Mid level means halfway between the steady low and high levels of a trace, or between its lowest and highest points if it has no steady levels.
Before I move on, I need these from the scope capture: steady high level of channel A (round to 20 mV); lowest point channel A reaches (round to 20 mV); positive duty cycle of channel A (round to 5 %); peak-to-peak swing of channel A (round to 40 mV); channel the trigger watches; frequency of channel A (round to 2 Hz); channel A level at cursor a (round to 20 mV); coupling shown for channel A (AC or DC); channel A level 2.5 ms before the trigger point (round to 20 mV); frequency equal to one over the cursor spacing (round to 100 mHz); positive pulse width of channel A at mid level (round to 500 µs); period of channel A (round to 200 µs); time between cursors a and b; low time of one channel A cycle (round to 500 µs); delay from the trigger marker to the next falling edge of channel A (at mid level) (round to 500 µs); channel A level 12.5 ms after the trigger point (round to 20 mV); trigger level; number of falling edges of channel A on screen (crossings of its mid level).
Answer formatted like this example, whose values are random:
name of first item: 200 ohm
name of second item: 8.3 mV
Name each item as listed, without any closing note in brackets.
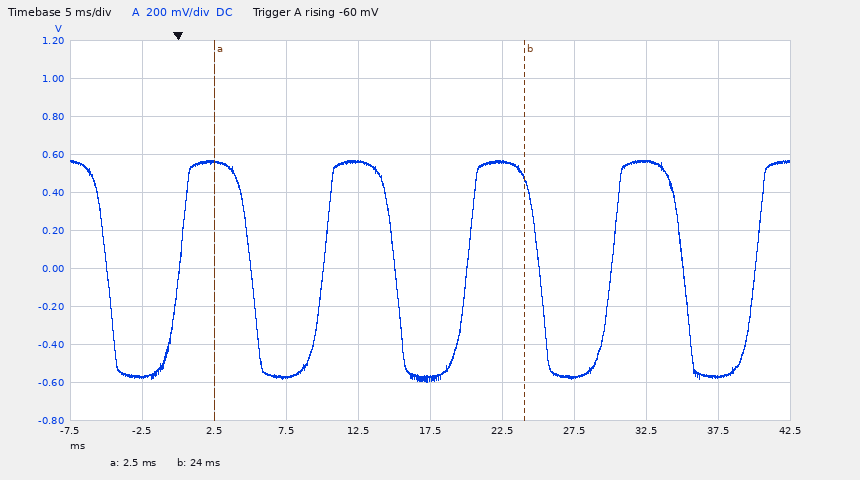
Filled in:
steady high level of channel A: 560 mV
lowest point channel A reaches: -600 mV
positive duty cycle of channel A: 50 %
peak-to-peak swing of channel A: 1.16 V
channel the trigger watches: channel A
frequency of channel A: 100 Hz
channel A level at cursor a: 560 mV
coupling shown for channel A: DC
channel A level 2.5 ms before the trigger point: -580 mV
frequency equal to one over the cursor spacing: 46.5 Hz
positive pulse width of channel A at mid level: 5.0 ms
period of channel A: 10.0 ms
time between cursors a and b: 21.5 ms
low time of one channel A cycle: 5.0 ms
delay from the trigger marker to the next falling edge of channel A (at mid level): 5.0 ms
channel A level 12.5 ms after the trigger point: 560 mV
trigger level: -60 mV
number of falling edges of channel A on screen: 5
